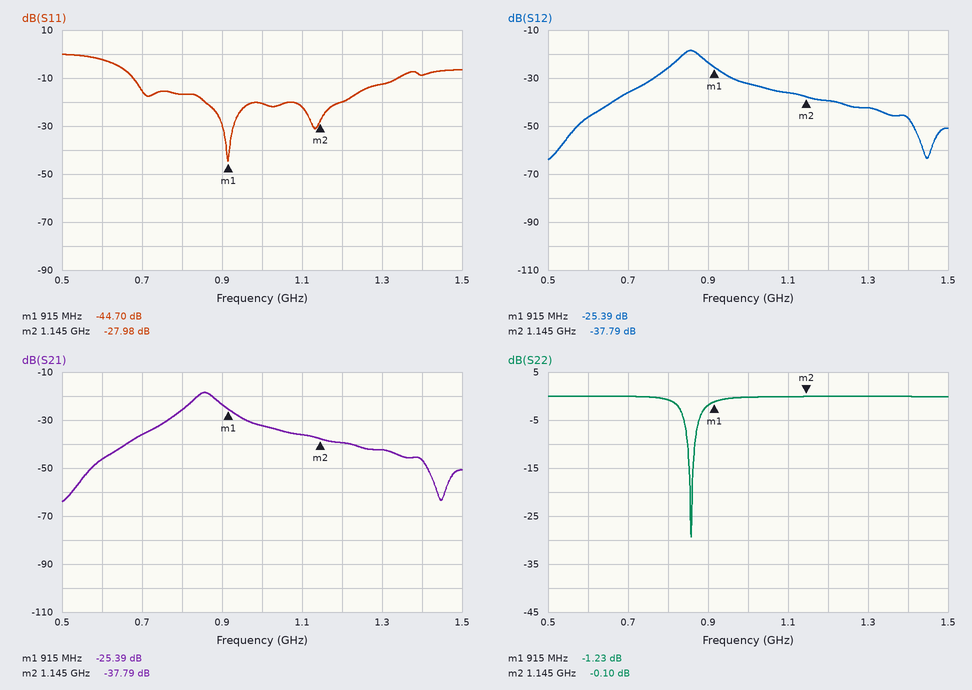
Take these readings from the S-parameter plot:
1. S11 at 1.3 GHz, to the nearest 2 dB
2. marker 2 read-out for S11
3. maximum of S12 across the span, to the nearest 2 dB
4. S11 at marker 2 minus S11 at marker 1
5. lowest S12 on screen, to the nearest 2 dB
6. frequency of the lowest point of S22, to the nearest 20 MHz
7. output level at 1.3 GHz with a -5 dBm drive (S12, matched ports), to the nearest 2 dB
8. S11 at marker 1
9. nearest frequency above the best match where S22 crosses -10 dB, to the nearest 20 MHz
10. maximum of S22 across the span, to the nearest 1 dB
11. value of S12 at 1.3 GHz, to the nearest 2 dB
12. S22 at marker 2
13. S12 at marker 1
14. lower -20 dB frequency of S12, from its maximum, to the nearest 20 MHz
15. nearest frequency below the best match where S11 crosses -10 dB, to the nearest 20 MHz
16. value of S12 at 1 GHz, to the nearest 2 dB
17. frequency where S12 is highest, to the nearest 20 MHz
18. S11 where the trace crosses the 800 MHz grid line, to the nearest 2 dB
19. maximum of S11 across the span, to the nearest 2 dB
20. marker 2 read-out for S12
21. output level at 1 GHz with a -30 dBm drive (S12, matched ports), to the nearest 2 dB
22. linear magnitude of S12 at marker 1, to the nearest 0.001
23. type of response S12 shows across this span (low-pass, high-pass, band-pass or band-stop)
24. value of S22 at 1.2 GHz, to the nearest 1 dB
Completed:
-12 dB
-27.98 dB
-18 dB
16.72 dB
-64 dB
860 MHz
-48 dBm
-44.70 dB
860 MHz
0 dB
-42 dB
-0.10 dB
-25.39 dB
680 MHz
680 MHz
-32 dB
860 MHz
-16 dB
0 dB
-37.79 dB
-62 dBm
0.054
band-pass
0 dB
